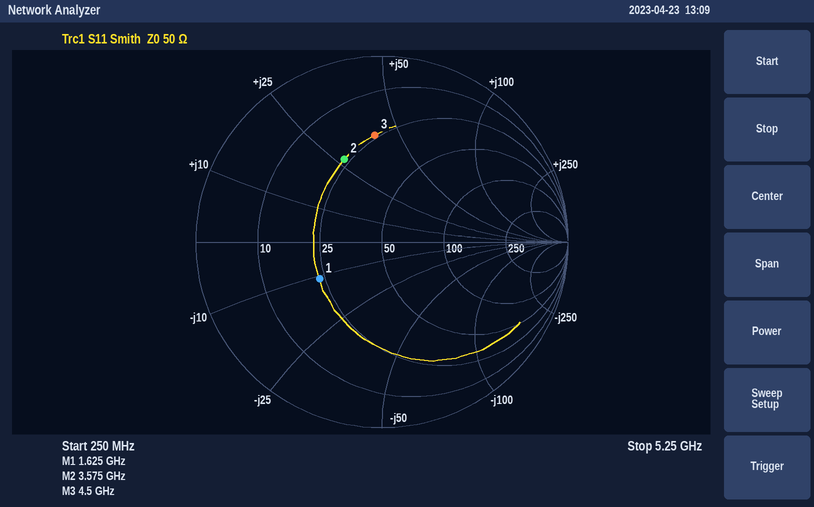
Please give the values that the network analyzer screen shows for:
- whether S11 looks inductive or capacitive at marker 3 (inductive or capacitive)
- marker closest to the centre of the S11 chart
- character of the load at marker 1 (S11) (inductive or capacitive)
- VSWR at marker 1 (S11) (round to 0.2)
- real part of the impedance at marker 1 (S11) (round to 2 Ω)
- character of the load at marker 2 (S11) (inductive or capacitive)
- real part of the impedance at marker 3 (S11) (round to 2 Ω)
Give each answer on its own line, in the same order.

inductive
marker 1
capacitive
2.2
24 Ω
inductive
24 Ω
